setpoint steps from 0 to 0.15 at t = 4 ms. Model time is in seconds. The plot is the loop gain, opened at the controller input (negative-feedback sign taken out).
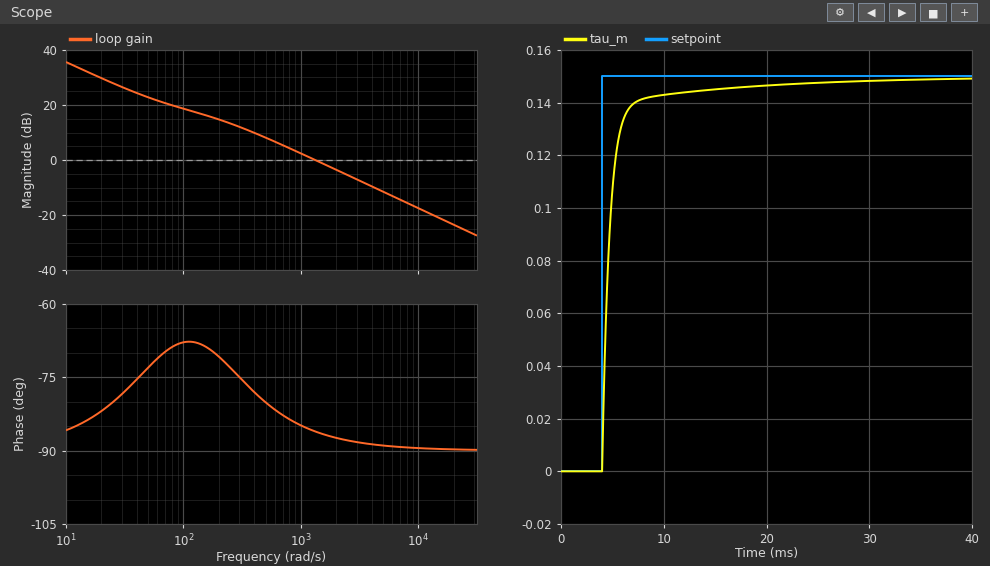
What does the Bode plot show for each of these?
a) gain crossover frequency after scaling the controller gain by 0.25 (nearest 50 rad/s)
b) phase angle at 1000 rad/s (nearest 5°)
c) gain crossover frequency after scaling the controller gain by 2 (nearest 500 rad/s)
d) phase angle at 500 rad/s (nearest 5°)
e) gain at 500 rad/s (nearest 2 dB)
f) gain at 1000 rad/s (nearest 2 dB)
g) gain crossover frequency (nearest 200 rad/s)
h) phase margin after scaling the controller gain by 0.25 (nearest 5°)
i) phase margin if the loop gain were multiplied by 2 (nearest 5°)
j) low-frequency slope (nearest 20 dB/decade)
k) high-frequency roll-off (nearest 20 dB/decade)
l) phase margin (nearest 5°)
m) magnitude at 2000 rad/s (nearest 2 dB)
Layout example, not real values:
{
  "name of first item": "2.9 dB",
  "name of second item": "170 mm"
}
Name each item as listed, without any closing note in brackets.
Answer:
{
  "gain crossover frequency after scaling the controller gain by 0.25": "300 rad/s",
  "phase angle at 1000 rad/s": "-85°",
  "gain crossover frequency after scaling the controller gain by 2": "2500 rad/s",
  "phase angle at 500 rad/s": "-80°",
  "gain at 500 rad/s": "8 dB",
  "gain at 1000 rad/s": "2 dB",
  "gain crossover frequency": "1400 rad/s",
  "phase margin after scaling the controller gain by 0.25": "105°",
  "phase margin if the loop gain were multiplied by 2": "90°",
  "low-frequency slope": "-20 dB/decade",
  "high-frequency roll-off": "-20 dB/decade",
  "phase margin": "95°",
  "magnitude at 2000 rad/s": "-4 dB"
}
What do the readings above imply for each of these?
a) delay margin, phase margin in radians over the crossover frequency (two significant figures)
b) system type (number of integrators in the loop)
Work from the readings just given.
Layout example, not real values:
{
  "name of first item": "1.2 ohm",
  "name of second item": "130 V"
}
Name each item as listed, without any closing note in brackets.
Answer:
{
  "delay margin, phase margin in radians over the crossover frequency": "0.0012 s",
  "system type": "1"
}
